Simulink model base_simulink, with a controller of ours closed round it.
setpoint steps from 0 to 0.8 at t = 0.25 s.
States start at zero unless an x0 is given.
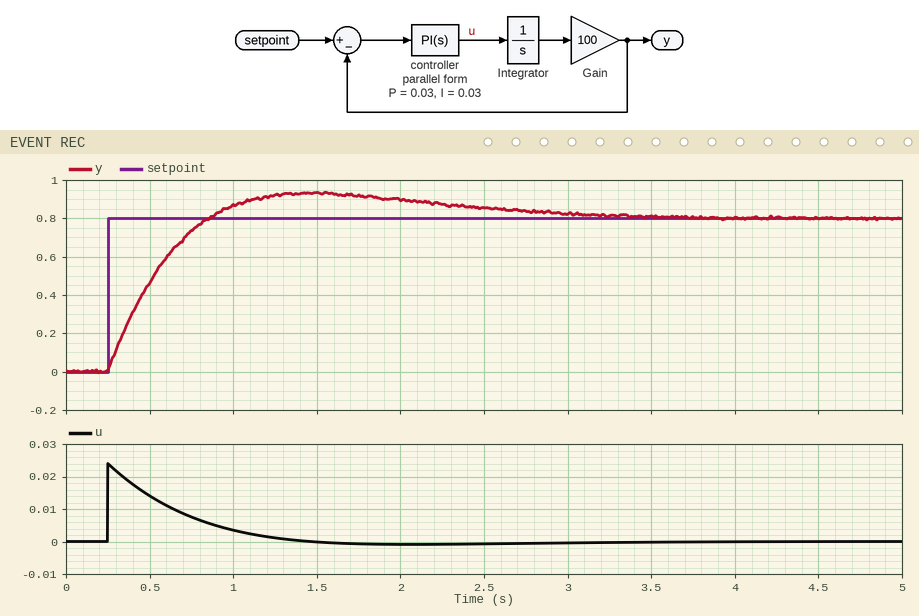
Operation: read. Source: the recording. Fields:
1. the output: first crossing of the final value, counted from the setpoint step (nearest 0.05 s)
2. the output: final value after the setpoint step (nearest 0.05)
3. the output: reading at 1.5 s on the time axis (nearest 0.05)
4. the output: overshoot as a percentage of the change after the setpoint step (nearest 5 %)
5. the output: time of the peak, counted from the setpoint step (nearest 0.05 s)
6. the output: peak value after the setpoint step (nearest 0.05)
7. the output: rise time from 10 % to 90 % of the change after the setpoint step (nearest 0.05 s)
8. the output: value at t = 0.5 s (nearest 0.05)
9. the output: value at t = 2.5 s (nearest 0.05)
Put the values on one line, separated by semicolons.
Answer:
0.60 s; 0.80; 0.95; 15 %; 1.20 s; 0.95; 0.45 s; 0.45; 0.85
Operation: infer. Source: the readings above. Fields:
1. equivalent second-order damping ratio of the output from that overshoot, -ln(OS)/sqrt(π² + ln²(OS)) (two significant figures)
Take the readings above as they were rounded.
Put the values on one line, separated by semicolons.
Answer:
0.52
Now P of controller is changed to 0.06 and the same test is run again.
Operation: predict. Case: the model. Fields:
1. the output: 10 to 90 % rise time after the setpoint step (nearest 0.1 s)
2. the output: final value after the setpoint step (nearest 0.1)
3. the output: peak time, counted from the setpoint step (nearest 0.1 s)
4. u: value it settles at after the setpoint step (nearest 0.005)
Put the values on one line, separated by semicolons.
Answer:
0.3 s; 0.8; 0.9 s; 0.000
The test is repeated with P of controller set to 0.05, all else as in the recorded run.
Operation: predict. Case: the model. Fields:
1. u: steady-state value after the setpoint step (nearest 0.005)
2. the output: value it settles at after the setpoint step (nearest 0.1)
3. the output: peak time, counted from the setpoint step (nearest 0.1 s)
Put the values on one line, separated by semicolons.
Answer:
0.000; 0.8; 1.0 s
